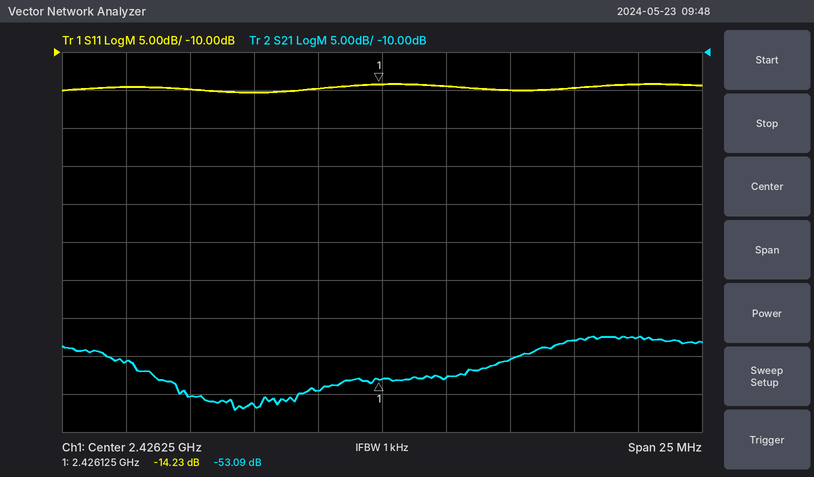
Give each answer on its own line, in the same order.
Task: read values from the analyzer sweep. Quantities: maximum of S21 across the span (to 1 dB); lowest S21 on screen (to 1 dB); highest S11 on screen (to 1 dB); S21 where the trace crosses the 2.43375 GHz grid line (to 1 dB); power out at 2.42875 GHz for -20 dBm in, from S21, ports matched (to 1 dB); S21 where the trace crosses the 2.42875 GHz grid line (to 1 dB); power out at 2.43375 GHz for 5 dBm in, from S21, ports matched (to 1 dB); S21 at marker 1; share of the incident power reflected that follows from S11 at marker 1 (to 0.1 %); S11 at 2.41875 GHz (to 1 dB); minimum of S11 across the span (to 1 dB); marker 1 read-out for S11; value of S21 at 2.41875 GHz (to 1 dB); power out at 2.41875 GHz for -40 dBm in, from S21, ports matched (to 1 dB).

-47 dB
-57 dB
-14 dB
-48 dB
-73 dBm
-53 dB
-43 dBm
-53.09 dB
3.8 %
-15 dB
-15 dB
-14.23 dB
-55 dB
-95 dBm
